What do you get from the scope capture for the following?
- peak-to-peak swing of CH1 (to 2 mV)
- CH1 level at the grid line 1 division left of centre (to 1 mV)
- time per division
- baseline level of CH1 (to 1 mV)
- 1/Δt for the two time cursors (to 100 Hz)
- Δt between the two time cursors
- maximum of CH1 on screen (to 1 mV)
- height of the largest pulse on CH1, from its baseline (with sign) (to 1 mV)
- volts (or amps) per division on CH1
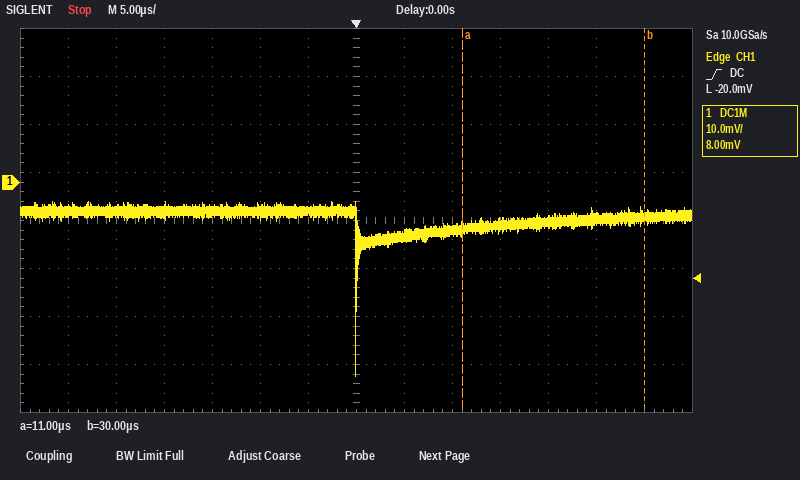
36 mV
-6 mV
5 µs
-6 mV
52.6 kHz
19.0 µs
-4 mV
-34 mV
10 mV
